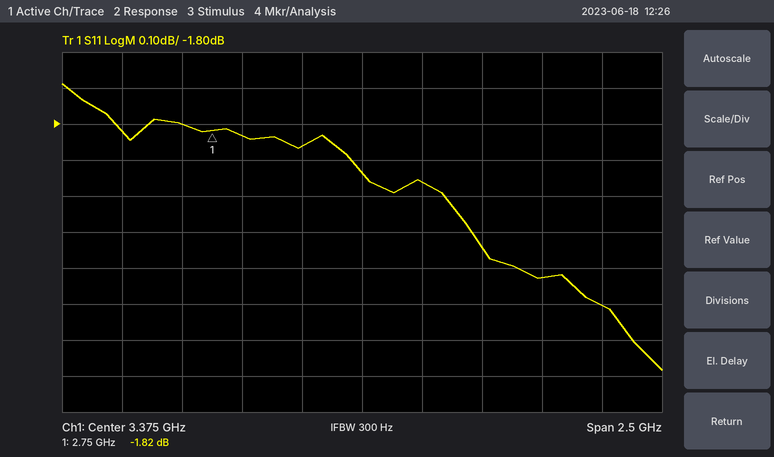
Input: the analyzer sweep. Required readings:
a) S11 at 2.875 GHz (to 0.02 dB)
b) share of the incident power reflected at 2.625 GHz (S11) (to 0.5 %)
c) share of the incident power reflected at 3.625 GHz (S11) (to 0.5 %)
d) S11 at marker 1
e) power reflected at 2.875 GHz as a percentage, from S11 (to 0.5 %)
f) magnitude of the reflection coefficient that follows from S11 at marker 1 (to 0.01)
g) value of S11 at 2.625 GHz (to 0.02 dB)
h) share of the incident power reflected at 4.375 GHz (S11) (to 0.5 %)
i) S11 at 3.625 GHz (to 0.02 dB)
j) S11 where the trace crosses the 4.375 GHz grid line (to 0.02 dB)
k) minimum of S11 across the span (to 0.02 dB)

-1.84 dB
66.0 %
63.5 %
-1.82 dB
65.5 %
0.81
-1.80 dB
59.0 %
-1.96 dB
-2.30 dB
-2.48 dB
